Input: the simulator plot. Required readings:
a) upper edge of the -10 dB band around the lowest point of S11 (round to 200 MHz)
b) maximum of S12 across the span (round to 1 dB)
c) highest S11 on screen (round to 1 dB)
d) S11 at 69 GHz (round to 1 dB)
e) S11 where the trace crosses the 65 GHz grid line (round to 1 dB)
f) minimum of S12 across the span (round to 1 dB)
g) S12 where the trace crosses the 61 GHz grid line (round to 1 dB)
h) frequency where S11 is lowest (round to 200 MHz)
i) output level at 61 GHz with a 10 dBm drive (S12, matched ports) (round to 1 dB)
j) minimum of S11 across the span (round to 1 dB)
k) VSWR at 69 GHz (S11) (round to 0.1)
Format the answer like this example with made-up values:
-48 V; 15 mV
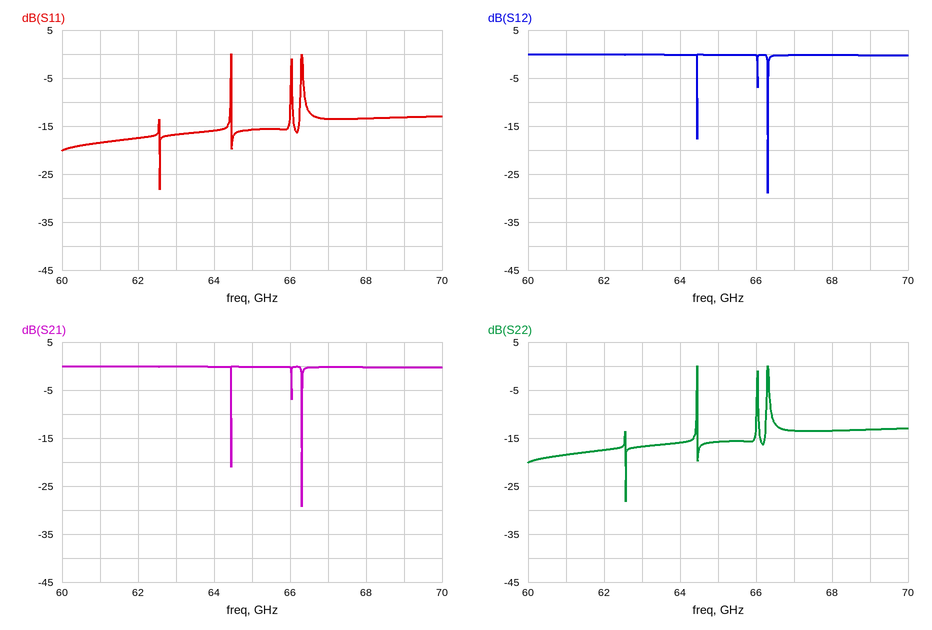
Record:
64.4 GHz; 0 dB; 0 dB; -13 dB; -16 dB; -29 dB; 0 dB; 62.6 GHz; 10 dBm; -28 dB; 1.6
